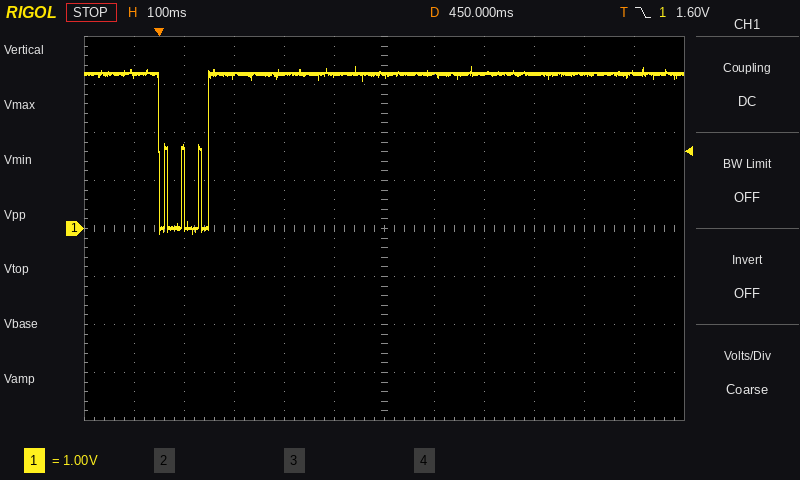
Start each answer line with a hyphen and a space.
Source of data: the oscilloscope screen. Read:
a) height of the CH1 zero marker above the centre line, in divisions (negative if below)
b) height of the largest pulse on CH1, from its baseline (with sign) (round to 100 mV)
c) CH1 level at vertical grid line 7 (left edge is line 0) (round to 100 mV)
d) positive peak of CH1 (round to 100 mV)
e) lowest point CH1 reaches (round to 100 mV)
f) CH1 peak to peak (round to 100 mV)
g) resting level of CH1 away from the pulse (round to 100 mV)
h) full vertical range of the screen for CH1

- 0.0 div
- -3.3 V
- 3.2 V
- 3.4 V
- -100 mV
- 3.5 V
- 3.2 V
- 8 V
